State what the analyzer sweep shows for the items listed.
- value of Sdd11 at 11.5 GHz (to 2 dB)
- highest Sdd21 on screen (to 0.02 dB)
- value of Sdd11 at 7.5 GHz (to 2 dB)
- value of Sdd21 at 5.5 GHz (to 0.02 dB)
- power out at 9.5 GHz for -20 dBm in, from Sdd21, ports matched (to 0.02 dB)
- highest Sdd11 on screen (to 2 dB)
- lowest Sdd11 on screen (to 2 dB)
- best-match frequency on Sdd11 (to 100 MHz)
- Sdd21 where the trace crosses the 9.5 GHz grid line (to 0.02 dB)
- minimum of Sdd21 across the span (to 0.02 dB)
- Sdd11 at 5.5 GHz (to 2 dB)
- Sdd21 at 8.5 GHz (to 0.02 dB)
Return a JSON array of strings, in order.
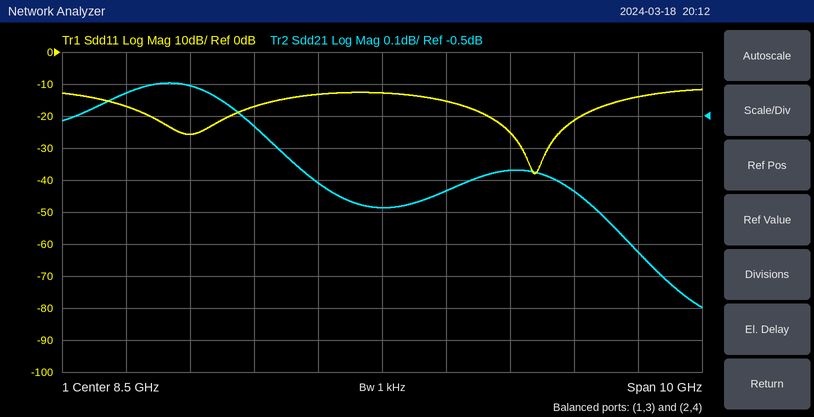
["-22 dB", "-0.40 dB", "-14 dB", "-0.40 dB", "-20.74 dBm", "-12 dB", "-38 dB", "10.9 GHz", "-0.74 dB", "-1.10 dB", "-26 dB", "-0.78 dB"]
